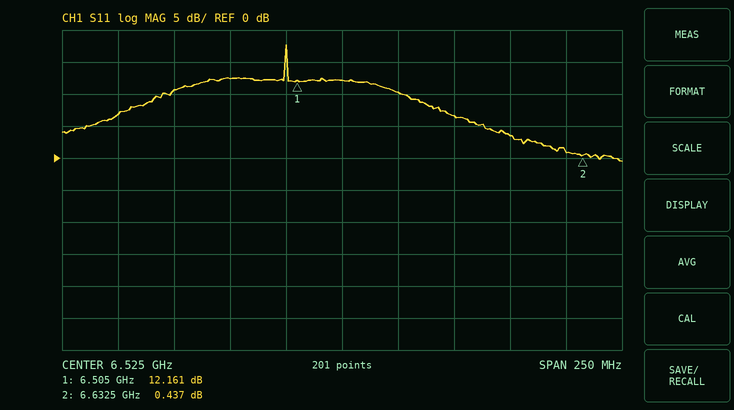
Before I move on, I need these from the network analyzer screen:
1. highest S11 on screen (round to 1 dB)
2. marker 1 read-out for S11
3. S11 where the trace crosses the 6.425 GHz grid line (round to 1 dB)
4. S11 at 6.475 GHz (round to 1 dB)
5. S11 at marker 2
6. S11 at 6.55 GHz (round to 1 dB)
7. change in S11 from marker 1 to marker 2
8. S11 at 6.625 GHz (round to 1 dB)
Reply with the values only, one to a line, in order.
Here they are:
18 dB
12.161 dB
7 dB
12 dB
0.437 dB
10 dB
-11.724 dB
1 dB
